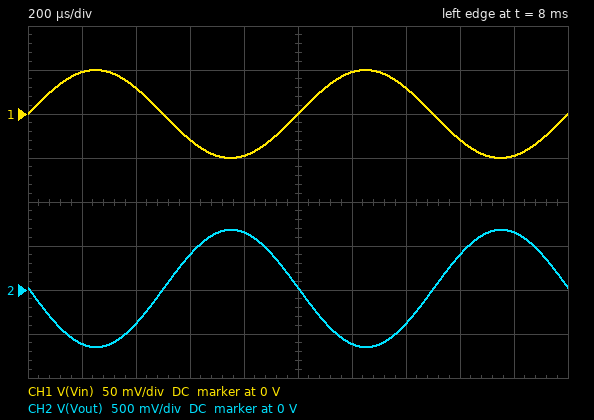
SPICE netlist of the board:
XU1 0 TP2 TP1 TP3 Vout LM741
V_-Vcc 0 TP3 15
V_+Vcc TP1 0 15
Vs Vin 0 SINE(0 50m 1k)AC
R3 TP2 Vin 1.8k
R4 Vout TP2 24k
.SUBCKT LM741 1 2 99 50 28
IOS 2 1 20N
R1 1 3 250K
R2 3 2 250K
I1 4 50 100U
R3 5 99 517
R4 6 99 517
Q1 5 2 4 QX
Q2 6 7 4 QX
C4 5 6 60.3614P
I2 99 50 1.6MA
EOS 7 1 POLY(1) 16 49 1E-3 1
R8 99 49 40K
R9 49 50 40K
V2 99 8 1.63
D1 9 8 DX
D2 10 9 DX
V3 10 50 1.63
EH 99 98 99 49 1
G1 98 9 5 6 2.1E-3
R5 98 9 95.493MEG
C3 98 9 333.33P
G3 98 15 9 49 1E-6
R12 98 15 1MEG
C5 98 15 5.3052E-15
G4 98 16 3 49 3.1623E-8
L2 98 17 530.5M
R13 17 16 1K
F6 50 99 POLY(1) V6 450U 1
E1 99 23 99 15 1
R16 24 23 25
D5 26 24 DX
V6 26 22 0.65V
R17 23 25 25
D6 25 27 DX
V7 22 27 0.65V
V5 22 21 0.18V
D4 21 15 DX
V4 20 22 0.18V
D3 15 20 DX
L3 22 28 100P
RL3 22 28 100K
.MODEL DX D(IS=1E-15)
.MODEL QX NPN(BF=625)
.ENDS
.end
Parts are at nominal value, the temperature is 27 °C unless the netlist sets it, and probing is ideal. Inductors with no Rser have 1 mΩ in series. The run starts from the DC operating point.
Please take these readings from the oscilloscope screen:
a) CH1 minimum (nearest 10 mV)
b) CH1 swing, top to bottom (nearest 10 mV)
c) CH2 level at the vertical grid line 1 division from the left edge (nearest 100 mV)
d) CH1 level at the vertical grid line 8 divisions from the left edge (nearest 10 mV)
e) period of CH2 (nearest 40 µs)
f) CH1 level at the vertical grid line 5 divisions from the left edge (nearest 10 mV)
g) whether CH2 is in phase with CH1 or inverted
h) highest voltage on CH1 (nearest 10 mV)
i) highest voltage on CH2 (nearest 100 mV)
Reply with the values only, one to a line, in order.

-50 mV
100 mV
-600 mV
-30 mV
1.00 ms
0 V
inverted
50 mV
700 mV
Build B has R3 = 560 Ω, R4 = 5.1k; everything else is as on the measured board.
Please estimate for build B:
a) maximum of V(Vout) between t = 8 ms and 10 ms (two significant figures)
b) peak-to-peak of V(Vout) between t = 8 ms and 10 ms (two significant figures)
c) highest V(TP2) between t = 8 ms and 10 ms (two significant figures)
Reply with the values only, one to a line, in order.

470 mV
910 mV
1.5 mV
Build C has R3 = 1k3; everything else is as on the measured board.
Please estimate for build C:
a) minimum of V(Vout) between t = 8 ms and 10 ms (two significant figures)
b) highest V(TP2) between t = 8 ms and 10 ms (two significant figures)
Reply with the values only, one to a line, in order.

-900 mV
1.9 mV
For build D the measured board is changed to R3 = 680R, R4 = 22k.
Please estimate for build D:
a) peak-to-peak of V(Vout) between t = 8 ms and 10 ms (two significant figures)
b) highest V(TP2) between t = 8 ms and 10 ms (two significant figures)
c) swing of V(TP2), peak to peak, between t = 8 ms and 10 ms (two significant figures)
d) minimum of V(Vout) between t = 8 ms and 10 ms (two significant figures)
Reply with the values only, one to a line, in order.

3.2 V
2.6 mV
3.3 mV
-1.6 V
